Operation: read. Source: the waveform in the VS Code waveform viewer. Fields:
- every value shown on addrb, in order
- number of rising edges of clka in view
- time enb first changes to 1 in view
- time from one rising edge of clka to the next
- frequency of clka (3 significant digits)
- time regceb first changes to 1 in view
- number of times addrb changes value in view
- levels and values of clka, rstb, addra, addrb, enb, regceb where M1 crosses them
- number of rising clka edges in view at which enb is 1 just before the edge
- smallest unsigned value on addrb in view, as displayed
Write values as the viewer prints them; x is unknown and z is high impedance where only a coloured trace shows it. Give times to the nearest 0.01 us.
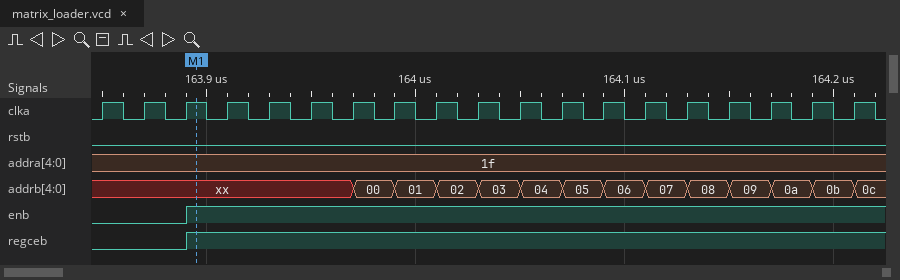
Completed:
xx, 00, 01, 02, 03, 04, 05, 06, 07, 08, 09, 0a, 0b, 0c
19
163.89 us
0.02 us
50.0 MHz
163.89 us
13
clka=1, rstb=0, addra=1f, addrb=xx, enb=1, regceb=1
16
00
